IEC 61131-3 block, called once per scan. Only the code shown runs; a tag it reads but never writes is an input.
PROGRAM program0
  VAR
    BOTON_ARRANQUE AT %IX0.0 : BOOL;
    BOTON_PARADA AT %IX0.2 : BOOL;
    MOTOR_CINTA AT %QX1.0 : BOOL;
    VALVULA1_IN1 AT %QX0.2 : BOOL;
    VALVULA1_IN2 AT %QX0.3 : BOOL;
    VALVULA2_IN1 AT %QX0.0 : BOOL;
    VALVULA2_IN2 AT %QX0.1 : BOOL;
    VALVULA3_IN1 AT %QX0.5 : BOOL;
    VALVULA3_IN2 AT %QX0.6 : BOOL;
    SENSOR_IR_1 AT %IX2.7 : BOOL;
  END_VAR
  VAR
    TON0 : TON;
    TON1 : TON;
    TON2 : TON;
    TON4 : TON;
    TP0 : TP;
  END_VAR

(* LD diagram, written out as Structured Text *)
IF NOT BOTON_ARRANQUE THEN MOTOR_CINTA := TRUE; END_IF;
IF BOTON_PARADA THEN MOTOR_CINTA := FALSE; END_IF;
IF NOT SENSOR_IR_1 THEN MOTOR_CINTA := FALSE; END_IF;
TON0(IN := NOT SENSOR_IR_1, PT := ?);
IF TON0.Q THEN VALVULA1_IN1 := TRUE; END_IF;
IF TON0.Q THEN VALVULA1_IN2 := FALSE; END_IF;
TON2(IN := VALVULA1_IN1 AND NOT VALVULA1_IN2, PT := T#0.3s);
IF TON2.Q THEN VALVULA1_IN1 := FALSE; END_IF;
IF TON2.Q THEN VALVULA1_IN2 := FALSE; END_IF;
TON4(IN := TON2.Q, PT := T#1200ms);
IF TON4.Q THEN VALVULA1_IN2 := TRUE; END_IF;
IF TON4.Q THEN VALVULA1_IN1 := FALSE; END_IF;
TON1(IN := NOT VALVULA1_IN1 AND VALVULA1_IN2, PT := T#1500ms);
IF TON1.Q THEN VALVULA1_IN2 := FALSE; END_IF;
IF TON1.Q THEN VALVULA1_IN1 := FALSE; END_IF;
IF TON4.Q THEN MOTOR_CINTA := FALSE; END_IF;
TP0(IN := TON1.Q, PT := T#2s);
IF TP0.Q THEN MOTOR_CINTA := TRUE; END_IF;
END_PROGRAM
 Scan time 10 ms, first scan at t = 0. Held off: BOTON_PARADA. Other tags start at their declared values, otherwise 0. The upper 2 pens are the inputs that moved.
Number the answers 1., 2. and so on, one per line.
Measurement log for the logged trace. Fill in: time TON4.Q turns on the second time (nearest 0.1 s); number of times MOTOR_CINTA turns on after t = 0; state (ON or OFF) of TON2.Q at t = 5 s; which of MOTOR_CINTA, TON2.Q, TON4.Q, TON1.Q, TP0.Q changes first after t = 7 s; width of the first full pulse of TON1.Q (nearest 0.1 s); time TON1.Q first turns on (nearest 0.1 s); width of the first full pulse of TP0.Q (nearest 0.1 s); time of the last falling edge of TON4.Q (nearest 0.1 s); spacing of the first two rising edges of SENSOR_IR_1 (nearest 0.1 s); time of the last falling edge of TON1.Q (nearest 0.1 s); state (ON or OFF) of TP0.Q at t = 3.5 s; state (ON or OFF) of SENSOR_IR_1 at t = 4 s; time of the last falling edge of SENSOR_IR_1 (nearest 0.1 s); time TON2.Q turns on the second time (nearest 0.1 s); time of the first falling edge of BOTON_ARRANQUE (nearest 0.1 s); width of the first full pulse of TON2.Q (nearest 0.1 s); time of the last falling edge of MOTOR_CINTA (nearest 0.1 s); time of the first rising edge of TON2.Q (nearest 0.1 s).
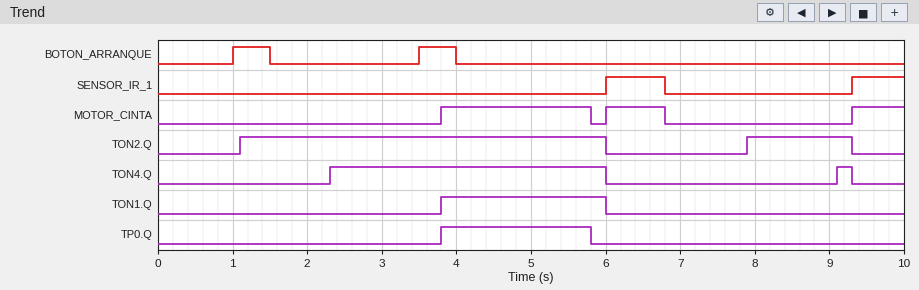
1. 9.1 s
2. 3
3. ON
4. TON2.Q
5. 2.2 s
6. 3.8 s
7. 2.0 s
8. 9.3 s
9. 3.3 s
10. 6.0 s
11. OFF
12. OFF
13. 6.8 s
14. 7.9 s
15. 1.5 s
16. 4.9 s
17. 6.8 s
18. 1.1 s
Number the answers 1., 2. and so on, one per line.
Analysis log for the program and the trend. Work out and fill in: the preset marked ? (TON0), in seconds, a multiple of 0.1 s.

1. 0.8 s
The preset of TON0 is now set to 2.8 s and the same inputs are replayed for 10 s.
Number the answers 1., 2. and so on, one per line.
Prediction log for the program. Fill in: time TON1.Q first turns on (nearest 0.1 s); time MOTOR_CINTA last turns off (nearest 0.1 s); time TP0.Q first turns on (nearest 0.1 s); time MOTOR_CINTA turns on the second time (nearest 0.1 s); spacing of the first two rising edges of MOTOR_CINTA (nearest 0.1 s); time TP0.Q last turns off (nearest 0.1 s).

1. 5.8 s
2. 7.8 s
3. 5.8 s
4. 9.3 s
5. 3.5 s
6. 7.8 s
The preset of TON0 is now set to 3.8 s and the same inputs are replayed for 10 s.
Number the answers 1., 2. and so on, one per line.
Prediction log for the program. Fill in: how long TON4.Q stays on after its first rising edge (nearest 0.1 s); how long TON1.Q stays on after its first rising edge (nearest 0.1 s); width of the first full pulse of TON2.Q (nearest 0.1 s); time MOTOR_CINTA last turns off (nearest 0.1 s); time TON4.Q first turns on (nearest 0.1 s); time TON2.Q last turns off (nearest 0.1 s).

1. 0.7 s
2. 0.0 s
3. 1.9 s
4. 8.8 s
5. 5.3 s
6. 6.0 s
